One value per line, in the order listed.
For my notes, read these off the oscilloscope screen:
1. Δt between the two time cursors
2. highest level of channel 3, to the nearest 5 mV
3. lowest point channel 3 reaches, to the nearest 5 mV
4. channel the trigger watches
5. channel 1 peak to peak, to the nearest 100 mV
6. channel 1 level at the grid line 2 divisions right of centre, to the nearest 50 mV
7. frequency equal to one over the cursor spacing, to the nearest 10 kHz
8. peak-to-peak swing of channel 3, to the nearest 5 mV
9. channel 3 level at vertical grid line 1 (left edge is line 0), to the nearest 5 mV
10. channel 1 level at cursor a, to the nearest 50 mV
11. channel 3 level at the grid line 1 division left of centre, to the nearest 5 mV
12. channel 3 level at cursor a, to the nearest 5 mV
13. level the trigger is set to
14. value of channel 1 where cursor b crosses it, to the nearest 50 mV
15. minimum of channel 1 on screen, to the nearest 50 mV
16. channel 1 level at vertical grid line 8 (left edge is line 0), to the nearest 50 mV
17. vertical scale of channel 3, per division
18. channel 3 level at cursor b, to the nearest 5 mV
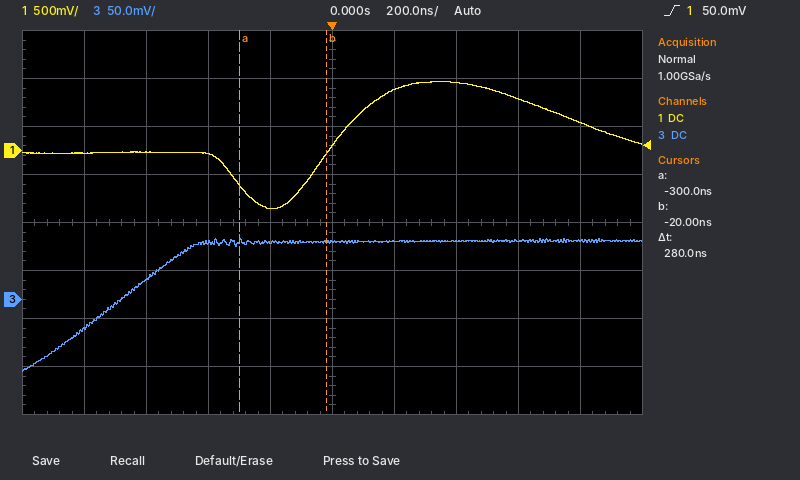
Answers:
280 ns
65 mV
-75 mV
channel 1
1.30 V
700 mV
3.57 MHz
140 mV
-30 mV
-350 mV
60 mV
60 mV
50.0 mV
-50 mV
-600 mV
550 mV
50 mV
60 mV
